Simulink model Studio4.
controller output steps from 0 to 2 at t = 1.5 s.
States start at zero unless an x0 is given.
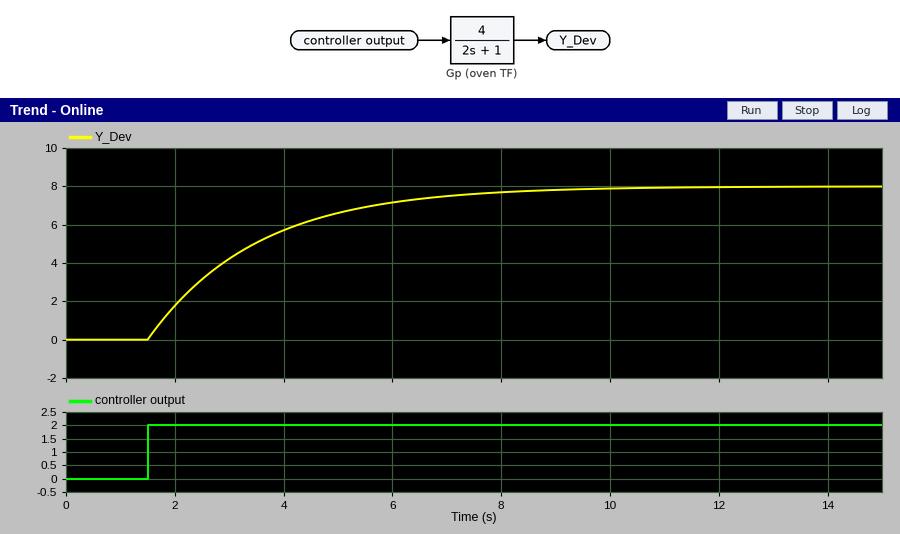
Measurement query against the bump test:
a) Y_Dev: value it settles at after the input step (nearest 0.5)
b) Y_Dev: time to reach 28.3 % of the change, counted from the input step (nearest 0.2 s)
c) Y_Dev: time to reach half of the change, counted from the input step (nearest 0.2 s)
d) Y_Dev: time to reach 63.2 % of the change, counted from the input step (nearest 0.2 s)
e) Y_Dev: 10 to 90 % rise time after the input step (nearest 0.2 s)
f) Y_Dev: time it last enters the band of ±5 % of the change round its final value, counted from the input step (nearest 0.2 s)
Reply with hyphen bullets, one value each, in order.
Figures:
- 8.0
- 0.6 s
- 1.4 s
- 2.0 s
- 4.4 s
- 6.0 s
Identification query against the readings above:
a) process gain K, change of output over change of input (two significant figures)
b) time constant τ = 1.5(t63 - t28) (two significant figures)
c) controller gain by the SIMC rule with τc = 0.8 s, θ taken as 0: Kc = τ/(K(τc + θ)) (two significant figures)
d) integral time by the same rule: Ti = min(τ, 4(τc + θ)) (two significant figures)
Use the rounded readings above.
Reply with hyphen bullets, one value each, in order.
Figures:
- 4.0
- 2.1 s
- 0.66
- 2.1 s
